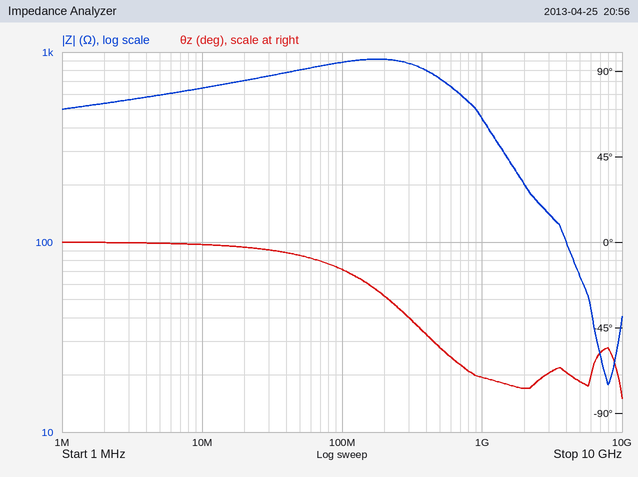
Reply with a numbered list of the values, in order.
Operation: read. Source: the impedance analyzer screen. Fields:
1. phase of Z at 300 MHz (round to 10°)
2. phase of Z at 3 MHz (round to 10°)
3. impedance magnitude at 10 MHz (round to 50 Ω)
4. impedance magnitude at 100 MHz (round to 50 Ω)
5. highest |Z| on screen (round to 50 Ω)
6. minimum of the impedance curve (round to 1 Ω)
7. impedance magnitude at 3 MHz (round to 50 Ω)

1. -40°
2. 0°
3. 650 Ω
4. 900 Ω
5. 900 Ω
6. 18 Ω
7. 550 Ω
